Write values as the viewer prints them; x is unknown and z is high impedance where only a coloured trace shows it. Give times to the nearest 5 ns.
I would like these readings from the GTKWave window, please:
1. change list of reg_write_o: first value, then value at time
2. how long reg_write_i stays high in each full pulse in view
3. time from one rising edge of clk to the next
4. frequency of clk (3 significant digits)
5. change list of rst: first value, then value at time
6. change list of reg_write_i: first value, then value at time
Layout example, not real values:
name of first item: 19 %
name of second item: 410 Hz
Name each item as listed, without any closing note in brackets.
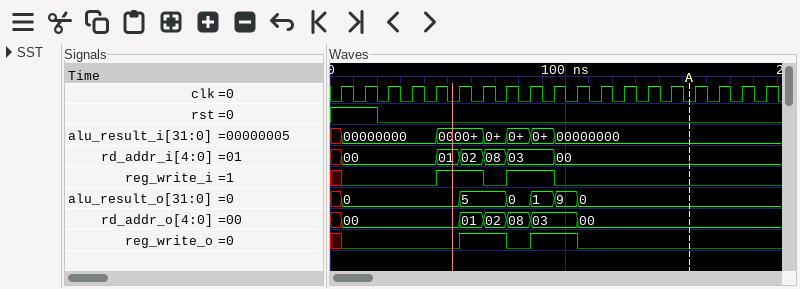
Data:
change list of reg_write_o: first value, then value at time: x, 0 at 5 ns, 1 at 55 ns, 0 at 75 ns, 1 at 85 ns, 0 at 105 ns
how long reg_write_i stays high in each full pulse in view: 20 ns, 20 ns
time from one rising edge of clk to the next: 10 ns
frequency of clk: 100 MHz
change list of rst: first value, then value at time: 1, 0 at 20 ns
change list of reg_write_i: first value, then value at time: x, 0 at 5 ns, 1 at 45 ns, 0 at 65 ns, 1 at 75 ns, 0 at 95 ns
